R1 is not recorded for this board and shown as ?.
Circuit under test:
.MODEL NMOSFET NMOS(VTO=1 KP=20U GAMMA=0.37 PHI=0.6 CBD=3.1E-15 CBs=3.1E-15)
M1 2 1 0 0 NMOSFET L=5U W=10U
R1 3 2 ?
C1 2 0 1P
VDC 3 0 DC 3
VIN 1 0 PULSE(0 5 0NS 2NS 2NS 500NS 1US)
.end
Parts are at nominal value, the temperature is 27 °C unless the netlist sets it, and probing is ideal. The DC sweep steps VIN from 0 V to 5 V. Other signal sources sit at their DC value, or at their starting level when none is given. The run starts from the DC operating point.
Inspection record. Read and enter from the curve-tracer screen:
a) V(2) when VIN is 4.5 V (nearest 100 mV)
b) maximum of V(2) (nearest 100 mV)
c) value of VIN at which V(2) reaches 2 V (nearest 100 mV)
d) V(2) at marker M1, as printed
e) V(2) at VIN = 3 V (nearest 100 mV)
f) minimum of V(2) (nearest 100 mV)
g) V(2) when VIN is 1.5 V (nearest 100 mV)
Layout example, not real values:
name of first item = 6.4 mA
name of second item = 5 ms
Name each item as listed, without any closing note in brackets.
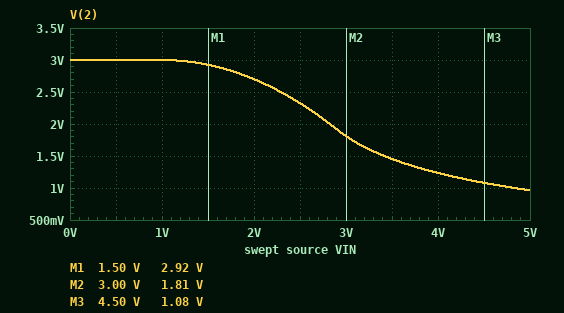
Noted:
V(2) when VIN is 4.5 V = 1.1 V
maximum of V(2) = 3.0 V
value of VIN at which V(2) reaches 2 V = 2.8 V
V(2) at marker M1, as printed = 2.92 V
V(2) at VIN = 3 V = 1.8 V
minimum of V(2) = 1.0 V
V(2) when VIN is 1.5 V = 2.9 V
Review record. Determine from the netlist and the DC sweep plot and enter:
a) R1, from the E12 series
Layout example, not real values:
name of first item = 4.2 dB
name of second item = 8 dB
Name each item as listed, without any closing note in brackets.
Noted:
R1, from the E12 series = 15 kΩ
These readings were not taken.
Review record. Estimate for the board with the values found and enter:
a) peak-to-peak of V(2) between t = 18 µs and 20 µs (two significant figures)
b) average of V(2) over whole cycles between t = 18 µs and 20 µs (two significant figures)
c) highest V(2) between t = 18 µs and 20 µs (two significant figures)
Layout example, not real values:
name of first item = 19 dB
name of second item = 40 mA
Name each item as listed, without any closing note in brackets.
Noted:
peak-to-peak of V(2) between t = 18 µs and 20 µs = 2.0 V
average of V(2) over whole cycles between t = 18 µs and 20 µs = 2.0 V
highest V(2) between t = 18 µs and 20 µs = 3.0 V
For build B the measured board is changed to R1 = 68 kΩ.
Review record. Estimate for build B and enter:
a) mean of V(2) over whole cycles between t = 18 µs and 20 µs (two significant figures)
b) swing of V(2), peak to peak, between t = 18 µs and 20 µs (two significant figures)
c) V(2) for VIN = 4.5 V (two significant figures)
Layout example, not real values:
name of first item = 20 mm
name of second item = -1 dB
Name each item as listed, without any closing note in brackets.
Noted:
mean of V(2) over whole cycles between t = 18 µs and 20 µs = 1.5 V
swing of V(2), peak to peak, between t = 18 µs and 20 µs = 2.7 V
V(2) for VIN = 4.5 V = 300 mV
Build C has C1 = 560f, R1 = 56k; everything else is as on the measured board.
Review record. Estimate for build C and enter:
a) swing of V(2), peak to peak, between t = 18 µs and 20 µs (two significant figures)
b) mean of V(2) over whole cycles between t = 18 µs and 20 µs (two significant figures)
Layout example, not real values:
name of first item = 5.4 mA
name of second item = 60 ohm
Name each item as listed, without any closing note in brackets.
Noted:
swing of V(2), peak to peak, between t = 18 µs and 20 µs = 2.7 V
mean of V(2) over whole cycles between t = 18 µs and 20 µs = 1.6 V
